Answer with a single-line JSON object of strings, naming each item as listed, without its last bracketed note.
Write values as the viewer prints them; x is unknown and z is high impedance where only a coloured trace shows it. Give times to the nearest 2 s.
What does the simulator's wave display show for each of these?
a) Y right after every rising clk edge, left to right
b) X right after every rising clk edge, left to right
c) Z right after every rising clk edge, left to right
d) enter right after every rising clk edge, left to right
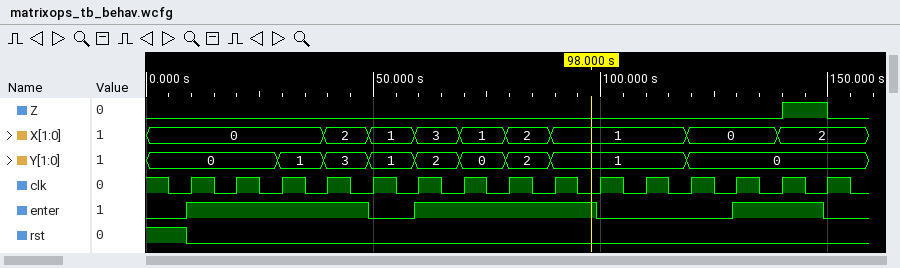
{"Y right after every rising clk edge, left to right": "0, 0, 1, 3, 1, 2, 0, 2, 1, 1, 1, 0, 0, 0, 0", "X right after every rising clk edge, left to right": "0, 0, 0, 2, 1, 3, 1, 2, 1, 1, 1, 0, 0, 2, 2", "Z right after every rising clk edge, left to right": "0 0 0 0 0 0 0 0 0 0 0 0 0 1 0", "enter right after every rising clk edge, left to right": "1 1 1 1 0 1 1 1 1 0 0 0 1 1 0"}
